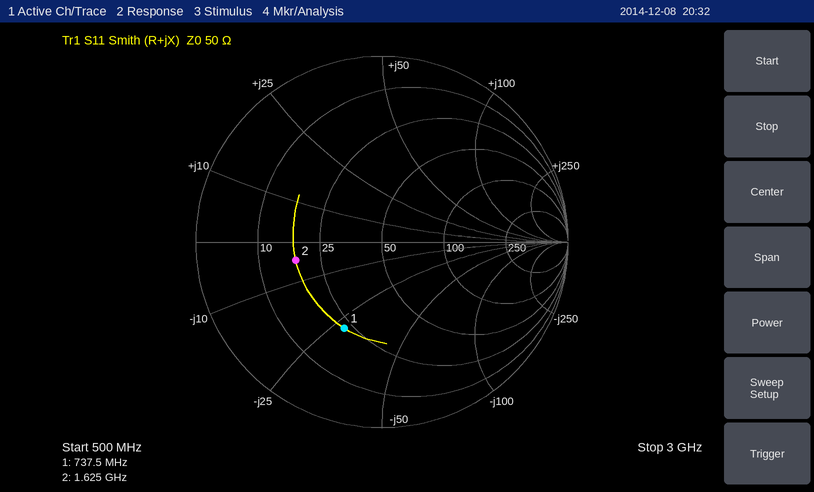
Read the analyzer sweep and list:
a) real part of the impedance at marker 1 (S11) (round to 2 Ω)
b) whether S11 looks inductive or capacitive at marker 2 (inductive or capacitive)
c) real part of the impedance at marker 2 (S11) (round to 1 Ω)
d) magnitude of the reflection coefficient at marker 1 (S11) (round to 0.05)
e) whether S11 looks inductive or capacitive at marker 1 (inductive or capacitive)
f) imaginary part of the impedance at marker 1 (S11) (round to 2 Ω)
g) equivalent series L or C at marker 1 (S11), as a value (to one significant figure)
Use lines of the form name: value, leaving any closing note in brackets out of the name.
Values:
real part of the impedance at marker 1 (S11): 22 Ω
whether S11 looks inductive or capacitive at marker 2: capacitive
real part of the impedance at marker 2 (S11): 18 Ω
magnitude of the reflection coefficient at marker 1 (S11): 0.50
whether S11 looks inductive or capacitive at marker 1: capacitive
imaginary part of the impedance at marker 1 (S11): -28 Ω
equivalent series L or C at marker 1 (S11), as a value: 8 pF
